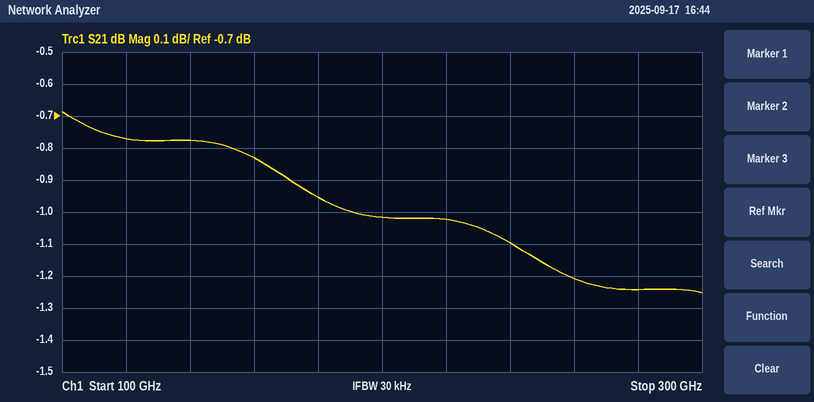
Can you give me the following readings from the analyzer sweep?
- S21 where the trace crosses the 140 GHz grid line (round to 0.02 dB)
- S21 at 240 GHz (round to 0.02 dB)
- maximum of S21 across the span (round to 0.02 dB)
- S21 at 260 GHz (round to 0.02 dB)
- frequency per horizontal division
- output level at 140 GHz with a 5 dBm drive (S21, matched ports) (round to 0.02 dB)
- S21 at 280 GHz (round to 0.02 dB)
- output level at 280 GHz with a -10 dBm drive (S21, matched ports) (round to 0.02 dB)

-0.78 dB
-1.10 dB
-0.68 dB
-1.20 dB
20 GHz
4.22 dBm
-1.24 dB
-11.24 dBm
